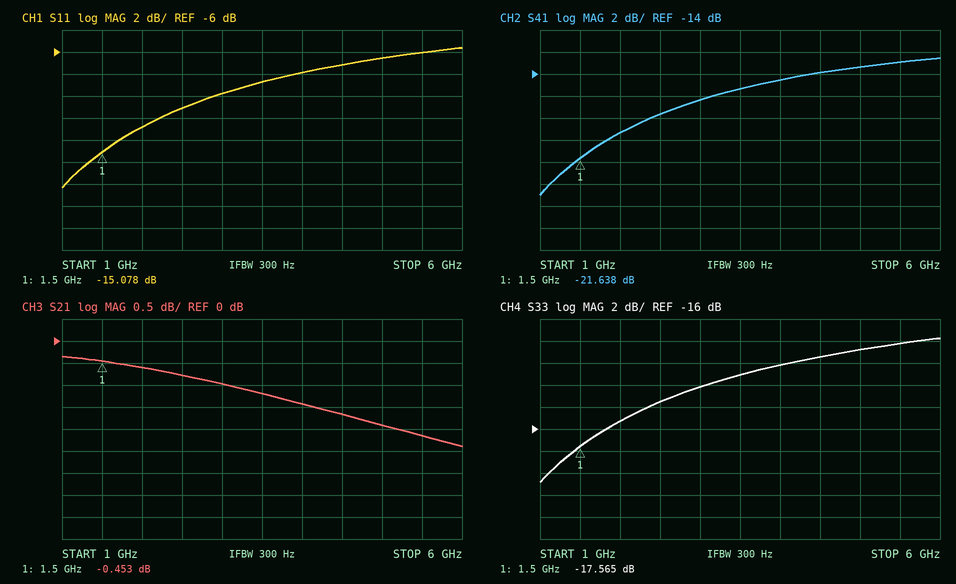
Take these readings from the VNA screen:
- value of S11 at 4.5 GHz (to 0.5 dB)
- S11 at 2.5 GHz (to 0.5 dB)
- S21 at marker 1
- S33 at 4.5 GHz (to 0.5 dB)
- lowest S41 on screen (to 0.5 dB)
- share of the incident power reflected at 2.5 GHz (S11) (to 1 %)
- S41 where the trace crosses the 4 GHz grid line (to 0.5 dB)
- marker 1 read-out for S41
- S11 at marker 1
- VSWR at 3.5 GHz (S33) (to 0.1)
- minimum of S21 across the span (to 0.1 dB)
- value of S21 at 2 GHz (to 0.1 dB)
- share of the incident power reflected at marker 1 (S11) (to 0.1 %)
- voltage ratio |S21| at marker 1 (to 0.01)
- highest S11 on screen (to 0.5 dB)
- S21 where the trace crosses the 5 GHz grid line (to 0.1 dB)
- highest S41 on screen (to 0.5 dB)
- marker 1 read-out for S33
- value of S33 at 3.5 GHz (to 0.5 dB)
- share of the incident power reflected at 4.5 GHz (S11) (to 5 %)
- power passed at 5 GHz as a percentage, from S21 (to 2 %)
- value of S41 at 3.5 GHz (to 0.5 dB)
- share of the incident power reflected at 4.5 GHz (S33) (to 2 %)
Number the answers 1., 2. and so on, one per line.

1. -7.0 dB
2. -11.0 dB
3. -0.453 dB
4. -9.5 dB
5. -25.0 dB
6. 8 %
7. -14.5 dB
8. -21.638 dB
9. -15.078 dB
10. 1.8
11. -2.4 dB
12. -0.6 dB
13. 3.1 %
14. 0.95
15. -5.5 dB
16. -1.9 dB
17. -12.5 dB
18. -17.565 dB
19. -11.0 dB
20. 20 %
21. 64 %
22. -15.5 dB
23. 12 %
